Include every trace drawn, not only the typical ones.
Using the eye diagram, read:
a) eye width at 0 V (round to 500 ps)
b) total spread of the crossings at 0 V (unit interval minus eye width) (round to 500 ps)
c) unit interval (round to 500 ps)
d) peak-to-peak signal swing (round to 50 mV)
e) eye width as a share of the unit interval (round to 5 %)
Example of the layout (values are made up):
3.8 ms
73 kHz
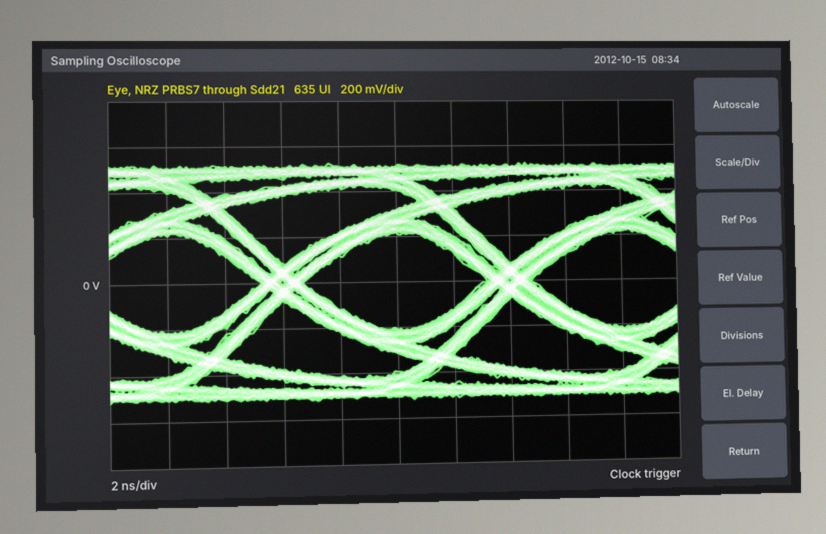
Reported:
6.5 ns
1.5 ns
8.0 ns
1.05 V
80 %
